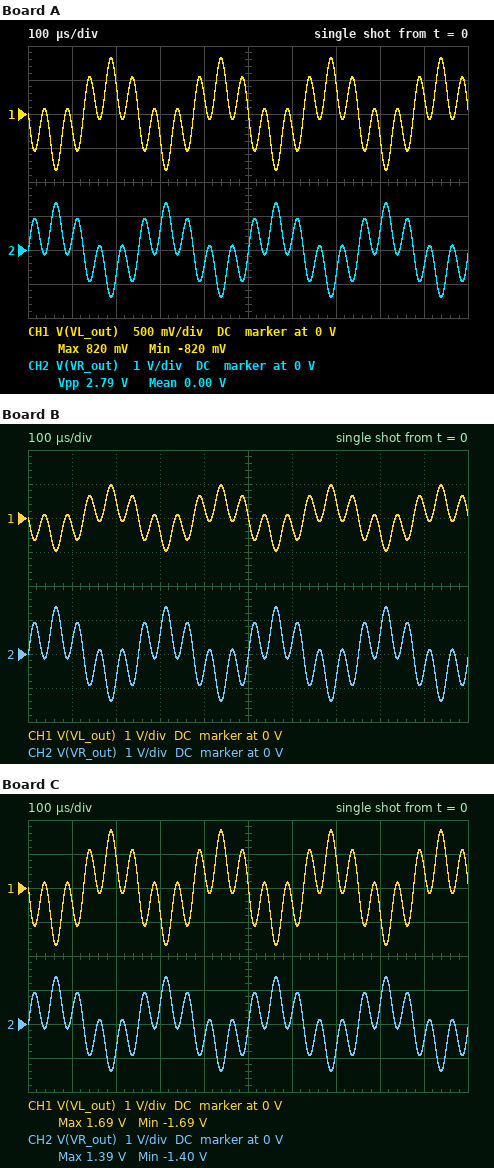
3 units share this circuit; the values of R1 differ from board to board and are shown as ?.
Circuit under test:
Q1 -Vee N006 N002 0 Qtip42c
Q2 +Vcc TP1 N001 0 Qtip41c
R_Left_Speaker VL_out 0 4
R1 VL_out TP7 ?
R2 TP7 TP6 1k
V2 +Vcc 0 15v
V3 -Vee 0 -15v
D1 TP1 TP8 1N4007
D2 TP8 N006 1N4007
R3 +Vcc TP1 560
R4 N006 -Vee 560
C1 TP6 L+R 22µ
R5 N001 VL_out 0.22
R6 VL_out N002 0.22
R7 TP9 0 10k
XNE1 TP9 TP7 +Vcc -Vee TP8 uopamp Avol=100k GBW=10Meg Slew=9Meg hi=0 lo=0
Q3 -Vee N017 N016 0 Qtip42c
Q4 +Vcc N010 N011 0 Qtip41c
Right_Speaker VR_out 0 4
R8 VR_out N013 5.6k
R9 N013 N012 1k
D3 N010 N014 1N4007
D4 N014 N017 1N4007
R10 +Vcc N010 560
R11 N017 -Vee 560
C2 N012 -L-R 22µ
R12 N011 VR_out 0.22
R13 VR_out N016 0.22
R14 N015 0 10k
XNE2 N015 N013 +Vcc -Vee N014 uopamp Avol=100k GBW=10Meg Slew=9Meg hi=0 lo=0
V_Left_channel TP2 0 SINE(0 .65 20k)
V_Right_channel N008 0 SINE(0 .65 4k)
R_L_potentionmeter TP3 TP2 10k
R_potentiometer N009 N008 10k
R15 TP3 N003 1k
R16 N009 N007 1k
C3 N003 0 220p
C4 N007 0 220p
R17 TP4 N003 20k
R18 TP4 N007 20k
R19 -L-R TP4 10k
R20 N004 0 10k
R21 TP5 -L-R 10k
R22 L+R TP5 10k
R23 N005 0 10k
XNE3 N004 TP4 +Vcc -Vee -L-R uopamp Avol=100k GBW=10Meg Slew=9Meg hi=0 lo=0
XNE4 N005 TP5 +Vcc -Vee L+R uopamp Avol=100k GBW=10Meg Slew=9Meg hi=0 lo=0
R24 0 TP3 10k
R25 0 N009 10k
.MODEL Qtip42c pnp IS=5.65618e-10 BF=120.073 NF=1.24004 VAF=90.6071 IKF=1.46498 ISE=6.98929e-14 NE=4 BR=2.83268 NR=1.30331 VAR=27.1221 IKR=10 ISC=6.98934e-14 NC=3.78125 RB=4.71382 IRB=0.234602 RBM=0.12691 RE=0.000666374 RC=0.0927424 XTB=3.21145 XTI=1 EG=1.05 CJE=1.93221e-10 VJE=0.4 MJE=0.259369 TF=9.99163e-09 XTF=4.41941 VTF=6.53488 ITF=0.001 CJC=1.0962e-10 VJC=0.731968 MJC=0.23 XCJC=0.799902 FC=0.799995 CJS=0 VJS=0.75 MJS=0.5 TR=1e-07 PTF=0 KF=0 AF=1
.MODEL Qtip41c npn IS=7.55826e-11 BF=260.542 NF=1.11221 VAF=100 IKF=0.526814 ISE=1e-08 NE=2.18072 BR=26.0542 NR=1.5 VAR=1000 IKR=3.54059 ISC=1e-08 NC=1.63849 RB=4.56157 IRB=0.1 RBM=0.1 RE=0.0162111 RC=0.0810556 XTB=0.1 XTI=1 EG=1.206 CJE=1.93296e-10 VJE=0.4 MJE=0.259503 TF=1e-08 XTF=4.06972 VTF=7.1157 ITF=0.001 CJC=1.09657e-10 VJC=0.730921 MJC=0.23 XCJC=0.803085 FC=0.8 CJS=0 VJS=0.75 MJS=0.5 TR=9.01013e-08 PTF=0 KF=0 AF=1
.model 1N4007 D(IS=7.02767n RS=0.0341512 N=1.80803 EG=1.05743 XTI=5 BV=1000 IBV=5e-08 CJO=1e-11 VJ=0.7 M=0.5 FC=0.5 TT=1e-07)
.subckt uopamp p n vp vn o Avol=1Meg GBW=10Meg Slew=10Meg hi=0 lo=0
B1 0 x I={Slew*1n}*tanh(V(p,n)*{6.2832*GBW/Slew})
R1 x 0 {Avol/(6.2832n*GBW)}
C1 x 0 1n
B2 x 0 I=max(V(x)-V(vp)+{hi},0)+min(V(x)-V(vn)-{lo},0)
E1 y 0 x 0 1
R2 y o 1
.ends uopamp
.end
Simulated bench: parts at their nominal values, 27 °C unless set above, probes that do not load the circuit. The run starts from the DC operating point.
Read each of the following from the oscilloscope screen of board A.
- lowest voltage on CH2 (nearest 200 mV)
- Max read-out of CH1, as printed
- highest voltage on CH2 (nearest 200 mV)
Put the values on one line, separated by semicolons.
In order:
-1.4 V; 820 mV; 1.4 V
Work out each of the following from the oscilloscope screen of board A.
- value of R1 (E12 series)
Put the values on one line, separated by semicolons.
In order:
3.3 kΩ
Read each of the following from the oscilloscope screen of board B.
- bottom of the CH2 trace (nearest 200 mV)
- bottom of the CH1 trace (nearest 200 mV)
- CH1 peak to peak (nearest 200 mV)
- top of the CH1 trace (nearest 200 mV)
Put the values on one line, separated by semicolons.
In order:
-1.4 V; -1.0 V; 2.0 V; 1.0 V
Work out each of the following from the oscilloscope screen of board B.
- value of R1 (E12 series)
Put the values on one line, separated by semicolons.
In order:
3.9 kΩ
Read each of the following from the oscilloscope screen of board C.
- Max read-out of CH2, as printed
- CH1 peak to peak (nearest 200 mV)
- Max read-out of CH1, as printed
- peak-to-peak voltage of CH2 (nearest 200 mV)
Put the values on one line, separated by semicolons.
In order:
1.39 V; 3.4 V; 1.69 V; 2.8 V
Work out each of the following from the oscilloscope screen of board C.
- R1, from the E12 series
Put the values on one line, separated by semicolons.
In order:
6.8 kΩ
